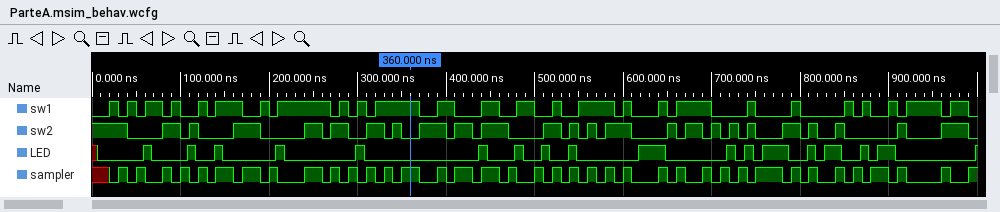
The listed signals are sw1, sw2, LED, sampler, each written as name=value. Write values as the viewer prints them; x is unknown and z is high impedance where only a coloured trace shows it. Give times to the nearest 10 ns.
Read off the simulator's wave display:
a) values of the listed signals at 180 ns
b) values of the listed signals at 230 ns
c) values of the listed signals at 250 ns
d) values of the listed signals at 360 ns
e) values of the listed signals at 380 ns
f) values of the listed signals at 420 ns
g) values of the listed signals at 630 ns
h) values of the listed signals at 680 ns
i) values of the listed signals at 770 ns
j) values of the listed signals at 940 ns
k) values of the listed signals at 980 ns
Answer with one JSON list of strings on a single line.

["sw1=0, sw2=1, LED=0, sampler=1", "sw1=1, sw2=0, LED=0, sampler=0", "sw1=1, sw2=1, LED=0, sampler=1", "sw1=1, sw2=0, LED=0, sampler=1", "sw1=0, sw2=1, LED=0, sampler=0", "sw1=0, sw2=1, LED=0, sampler=1", "sw1=0, sw2=0, LED=1, sampler=0", "sw1=1, sw2=1, LED=0, sampler=0", "sw1=0, sw2=0, LED=1, sampler=1", "sw1=1, sw2=0, LED=0, sampler=0", "sw1=1, sw2=1, LED=0, sampler=0"]
